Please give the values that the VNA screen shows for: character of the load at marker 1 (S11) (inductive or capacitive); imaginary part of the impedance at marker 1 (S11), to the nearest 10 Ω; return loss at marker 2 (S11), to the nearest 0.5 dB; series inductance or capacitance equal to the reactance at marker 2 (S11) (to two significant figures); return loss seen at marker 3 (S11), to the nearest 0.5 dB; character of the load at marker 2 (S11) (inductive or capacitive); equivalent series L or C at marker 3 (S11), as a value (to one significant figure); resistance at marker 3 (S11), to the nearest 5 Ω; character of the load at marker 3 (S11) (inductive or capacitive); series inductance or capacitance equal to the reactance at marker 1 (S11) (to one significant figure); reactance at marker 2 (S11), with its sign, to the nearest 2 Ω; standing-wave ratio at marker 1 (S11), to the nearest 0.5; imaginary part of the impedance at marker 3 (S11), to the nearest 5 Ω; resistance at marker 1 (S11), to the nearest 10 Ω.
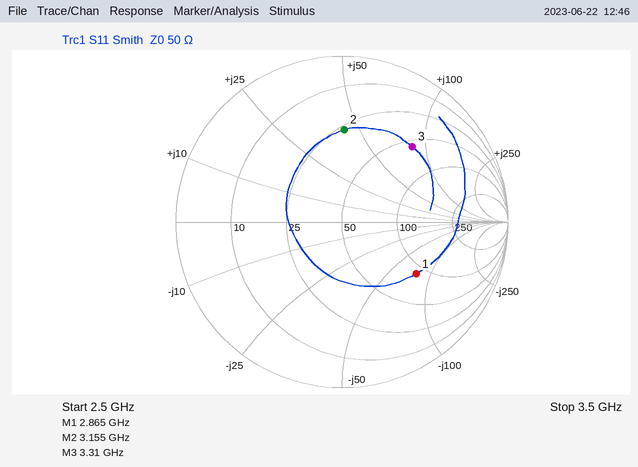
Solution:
capacitive
-80 Ω
5.0 dB
2.2 nH
4.0 dB
inductive
4 nH
55 Ω
inductive
700 fF
+44 Ω
3.5
+85 Ω
90 Ω
